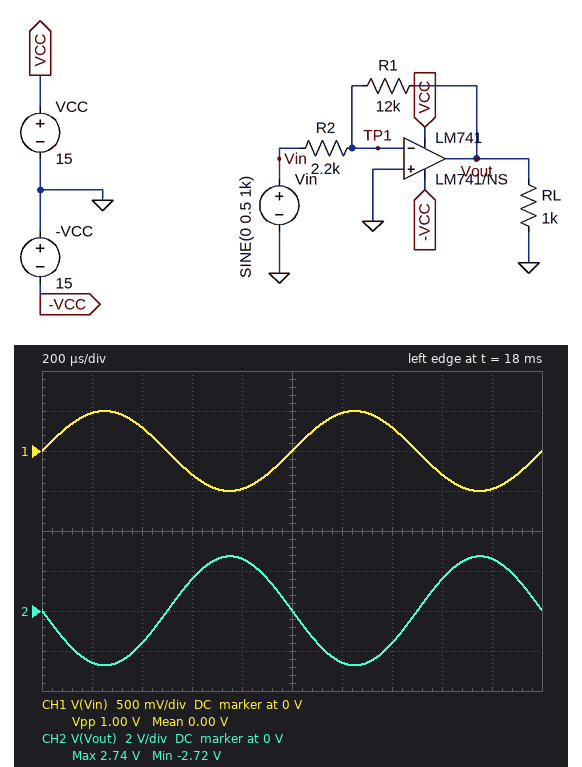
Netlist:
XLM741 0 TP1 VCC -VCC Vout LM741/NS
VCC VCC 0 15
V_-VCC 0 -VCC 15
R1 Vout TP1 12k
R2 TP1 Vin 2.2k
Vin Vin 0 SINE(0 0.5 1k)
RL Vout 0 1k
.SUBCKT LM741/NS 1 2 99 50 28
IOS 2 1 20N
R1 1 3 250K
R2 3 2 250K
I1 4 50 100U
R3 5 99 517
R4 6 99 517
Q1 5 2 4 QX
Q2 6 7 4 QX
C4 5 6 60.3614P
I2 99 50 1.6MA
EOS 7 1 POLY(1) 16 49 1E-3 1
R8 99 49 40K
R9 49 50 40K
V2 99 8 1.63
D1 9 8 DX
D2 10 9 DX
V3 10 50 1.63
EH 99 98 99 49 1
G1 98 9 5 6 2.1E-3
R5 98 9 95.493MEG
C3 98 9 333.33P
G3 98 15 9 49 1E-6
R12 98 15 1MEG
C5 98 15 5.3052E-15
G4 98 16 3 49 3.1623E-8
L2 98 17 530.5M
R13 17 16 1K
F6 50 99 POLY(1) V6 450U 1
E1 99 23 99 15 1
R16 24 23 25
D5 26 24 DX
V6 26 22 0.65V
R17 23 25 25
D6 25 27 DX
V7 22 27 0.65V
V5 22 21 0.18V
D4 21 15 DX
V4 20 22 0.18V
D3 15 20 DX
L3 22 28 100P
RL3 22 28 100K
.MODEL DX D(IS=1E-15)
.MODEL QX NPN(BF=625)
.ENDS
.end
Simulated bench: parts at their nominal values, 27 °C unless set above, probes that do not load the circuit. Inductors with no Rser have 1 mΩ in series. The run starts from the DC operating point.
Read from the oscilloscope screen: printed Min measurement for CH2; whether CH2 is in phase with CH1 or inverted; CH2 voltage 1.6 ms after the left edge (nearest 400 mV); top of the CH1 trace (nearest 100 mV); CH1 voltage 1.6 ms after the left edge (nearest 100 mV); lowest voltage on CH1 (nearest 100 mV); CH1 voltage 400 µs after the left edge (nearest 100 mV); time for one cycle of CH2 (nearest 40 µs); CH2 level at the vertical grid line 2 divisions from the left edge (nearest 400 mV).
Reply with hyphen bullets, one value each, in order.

- -2.72 V
- inverted
- 1.6 V
- 500 mV
- -300 mV
- -500 mV
- 300 mV
- 1.00 ms
- -1.6 V
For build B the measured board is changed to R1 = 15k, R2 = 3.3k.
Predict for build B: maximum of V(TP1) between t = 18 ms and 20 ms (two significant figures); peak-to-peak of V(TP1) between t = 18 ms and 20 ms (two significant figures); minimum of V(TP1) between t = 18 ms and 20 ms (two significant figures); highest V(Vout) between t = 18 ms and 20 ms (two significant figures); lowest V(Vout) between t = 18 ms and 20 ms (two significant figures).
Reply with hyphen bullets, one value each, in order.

- 3.7 mV
- 5.4 mV
- -1.7 mV
- 2.3 V
- -2.3 V
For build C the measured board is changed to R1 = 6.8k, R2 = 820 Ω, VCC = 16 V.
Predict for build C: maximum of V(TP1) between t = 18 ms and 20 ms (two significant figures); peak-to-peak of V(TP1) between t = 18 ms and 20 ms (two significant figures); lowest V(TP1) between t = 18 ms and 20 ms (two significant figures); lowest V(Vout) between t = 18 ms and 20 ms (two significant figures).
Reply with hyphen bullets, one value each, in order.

- 6.0 mV
- 10 mV
- -4.0 mV
- -4.1 V
